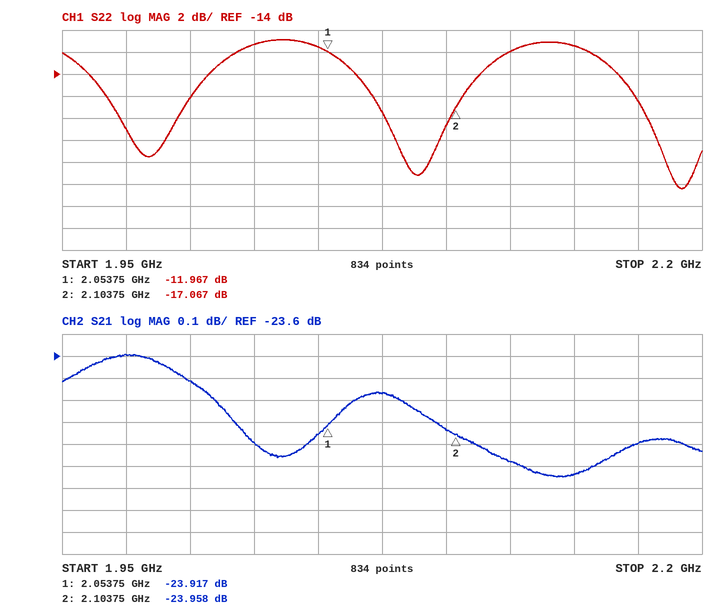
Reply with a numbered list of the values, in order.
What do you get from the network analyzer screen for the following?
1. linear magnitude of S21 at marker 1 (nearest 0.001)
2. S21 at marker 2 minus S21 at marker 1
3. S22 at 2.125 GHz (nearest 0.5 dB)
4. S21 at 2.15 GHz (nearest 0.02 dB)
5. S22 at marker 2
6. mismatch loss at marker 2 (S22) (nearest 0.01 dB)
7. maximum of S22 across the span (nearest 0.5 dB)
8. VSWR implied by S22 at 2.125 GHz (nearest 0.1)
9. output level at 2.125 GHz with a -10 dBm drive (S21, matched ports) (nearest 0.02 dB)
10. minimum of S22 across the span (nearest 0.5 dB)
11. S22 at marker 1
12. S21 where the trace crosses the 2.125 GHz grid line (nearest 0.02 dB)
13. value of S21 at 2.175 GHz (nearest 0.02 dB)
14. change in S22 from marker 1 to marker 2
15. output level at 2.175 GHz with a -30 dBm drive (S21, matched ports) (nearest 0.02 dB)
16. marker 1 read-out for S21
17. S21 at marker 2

1. 0.064
2. -0.041 dB
3. -12.0 dB
4. -24.14 dB
5. -17.067 dB
6. 0.09 dB
7. -11.0 dB
8. 1.7
9. -34.08 dBm
10. -24.5 dB
11. -11.967 dB
12. -24.08 dB
13. -24.00 dB
14. -5.100 dB
15. -54.00 dBm
16. -23.917 dB
17. -23.958 dB
